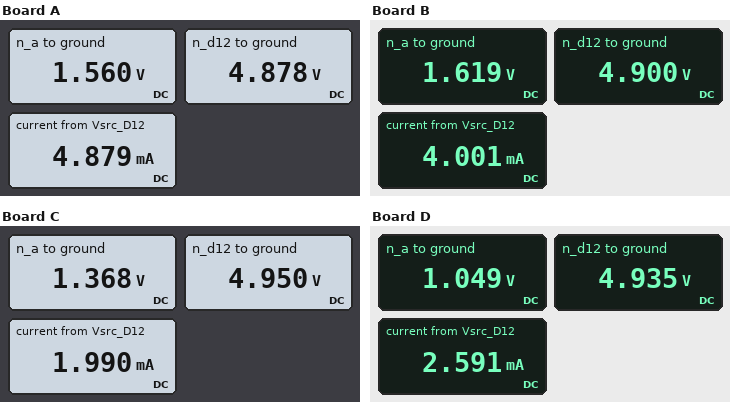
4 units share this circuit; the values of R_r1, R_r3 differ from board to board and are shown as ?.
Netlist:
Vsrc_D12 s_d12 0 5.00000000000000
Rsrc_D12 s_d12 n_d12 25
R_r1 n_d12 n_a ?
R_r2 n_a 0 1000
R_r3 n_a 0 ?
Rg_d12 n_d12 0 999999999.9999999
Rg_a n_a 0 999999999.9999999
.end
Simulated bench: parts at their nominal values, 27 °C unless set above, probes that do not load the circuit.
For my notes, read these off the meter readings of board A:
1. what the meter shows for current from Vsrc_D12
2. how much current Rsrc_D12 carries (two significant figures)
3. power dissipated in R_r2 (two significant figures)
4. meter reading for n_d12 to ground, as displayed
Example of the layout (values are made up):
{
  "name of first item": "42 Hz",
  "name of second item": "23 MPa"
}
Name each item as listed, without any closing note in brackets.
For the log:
{
  "what the meter shows for current from Vsrc_D12": "4.879 mA",
  "how much current Rsrc_D12 carries": "4.9 mA",
  "power dissipated in R_r2": "2.4 mW",
  "meter reading for n_d12 to ground, as displayed": "4.878 V"
}
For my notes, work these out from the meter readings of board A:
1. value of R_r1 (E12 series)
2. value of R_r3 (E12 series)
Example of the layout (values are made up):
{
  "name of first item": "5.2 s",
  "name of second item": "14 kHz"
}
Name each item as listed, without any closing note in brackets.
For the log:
{
  "value of R_r1": "680 Ω",
  "value of R_r3": "470 Ω"
}
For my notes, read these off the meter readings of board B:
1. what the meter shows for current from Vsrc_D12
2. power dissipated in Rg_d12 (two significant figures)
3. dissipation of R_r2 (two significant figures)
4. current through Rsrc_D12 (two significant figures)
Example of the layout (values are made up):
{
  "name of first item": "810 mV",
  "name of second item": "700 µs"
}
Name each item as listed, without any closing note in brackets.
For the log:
{
  "what the meter shows for current from Vsrc_D12": "4.001 mA",
  "power dissipated in Rg_d12": "24 nW",
  "dissipation of R_r2": "2.6 mW",
  "current through Rsrc_D12": "4.0 mA"
}
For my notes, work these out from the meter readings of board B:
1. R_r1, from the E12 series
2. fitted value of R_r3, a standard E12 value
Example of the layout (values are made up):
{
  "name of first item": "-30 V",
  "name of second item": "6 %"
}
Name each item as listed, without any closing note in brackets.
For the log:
{
  "R_r1, from the E12 series": "820 Ω",
  "fitted value of R_r3, a standard E12 value": "680 Ω"
}
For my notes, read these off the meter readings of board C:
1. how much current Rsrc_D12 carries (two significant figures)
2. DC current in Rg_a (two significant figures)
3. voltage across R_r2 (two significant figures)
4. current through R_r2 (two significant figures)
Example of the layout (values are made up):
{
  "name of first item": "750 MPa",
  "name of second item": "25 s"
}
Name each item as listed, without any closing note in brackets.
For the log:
{
  "how much current Rsrc_D12 carries": "2.0 mA",
  "DC current in Rg_a": "1.4 nA",
  "voltage across R_r2": "1.4 V",
  "current through R_r2": "1.4 mA"
}
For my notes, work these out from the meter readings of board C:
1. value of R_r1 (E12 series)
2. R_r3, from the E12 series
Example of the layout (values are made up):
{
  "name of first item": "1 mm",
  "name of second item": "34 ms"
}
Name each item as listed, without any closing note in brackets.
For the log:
{
  "value of R_r1": "1.8 kΩ",
  "R_r3, from the E12 series": "2.2 kΩ"
}
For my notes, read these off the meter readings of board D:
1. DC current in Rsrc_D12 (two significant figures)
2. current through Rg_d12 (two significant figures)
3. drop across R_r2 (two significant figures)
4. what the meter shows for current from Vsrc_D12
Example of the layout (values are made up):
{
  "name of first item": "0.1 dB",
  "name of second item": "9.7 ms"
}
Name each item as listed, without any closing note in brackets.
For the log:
{
  "DC current in Rsrc_D12": "2.6 mA",
  "current through Rg_d12": "4.9 nA",
  "drop across R_r2": "1.0 V",
  "what the meter shows for current from Vsrc_D12": "2.591 mA"
}
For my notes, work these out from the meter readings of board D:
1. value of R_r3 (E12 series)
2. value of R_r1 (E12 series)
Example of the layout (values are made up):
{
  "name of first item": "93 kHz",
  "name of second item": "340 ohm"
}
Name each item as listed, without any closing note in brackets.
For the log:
{
  "value of R_r3": "680 Ω",
  "value of R_r1": "1.5 kΩ"
}
